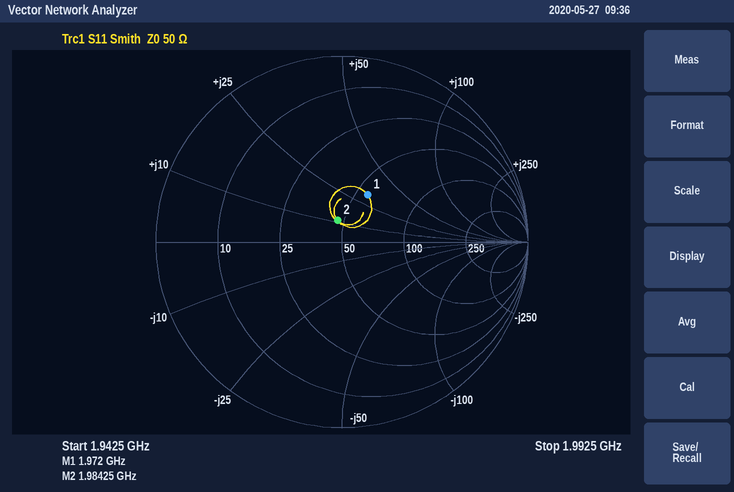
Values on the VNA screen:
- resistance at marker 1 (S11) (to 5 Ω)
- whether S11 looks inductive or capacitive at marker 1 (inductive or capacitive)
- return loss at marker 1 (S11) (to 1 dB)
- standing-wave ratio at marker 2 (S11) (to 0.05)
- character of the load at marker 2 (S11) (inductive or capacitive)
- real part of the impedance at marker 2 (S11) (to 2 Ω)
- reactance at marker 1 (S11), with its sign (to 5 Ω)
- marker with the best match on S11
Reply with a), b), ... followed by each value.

a) 55 Ω
b) inductive
c) 11 dB
d) 1.25
e) inductive
f) 46 Ω
g) +30 Ω
h) marker 2
